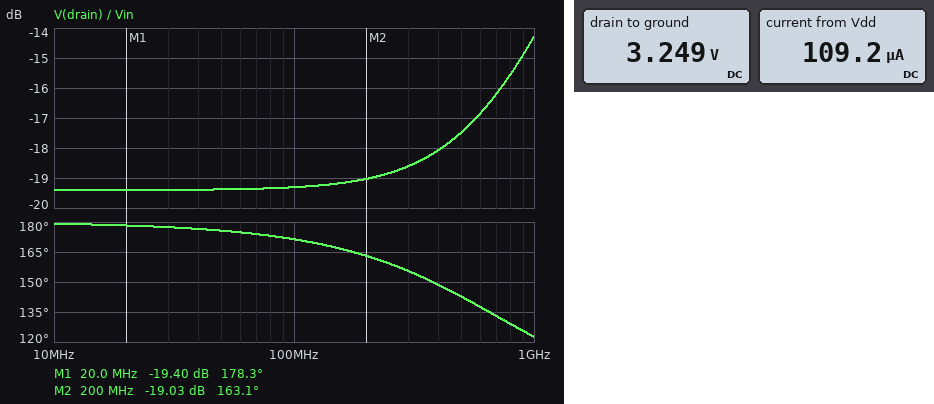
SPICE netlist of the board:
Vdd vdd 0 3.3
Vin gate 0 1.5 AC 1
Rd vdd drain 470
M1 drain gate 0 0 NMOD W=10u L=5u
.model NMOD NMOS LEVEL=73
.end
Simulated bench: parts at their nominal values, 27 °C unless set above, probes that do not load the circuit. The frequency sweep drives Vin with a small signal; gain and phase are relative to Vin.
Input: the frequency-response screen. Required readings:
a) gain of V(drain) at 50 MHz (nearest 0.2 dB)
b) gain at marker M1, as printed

-19.4 dB
-19.40 dB
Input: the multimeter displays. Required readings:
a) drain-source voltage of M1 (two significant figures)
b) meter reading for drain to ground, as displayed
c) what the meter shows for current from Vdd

3.2 V
3.249 V
109.2 µA
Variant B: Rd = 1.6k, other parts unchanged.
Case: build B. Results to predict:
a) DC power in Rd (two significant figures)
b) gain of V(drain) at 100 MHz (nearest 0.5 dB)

19 µW
-8.5 dB
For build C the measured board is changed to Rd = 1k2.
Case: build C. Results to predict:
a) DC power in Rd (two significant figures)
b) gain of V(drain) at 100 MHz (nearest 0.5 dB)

14 µW
-11.0 dB
